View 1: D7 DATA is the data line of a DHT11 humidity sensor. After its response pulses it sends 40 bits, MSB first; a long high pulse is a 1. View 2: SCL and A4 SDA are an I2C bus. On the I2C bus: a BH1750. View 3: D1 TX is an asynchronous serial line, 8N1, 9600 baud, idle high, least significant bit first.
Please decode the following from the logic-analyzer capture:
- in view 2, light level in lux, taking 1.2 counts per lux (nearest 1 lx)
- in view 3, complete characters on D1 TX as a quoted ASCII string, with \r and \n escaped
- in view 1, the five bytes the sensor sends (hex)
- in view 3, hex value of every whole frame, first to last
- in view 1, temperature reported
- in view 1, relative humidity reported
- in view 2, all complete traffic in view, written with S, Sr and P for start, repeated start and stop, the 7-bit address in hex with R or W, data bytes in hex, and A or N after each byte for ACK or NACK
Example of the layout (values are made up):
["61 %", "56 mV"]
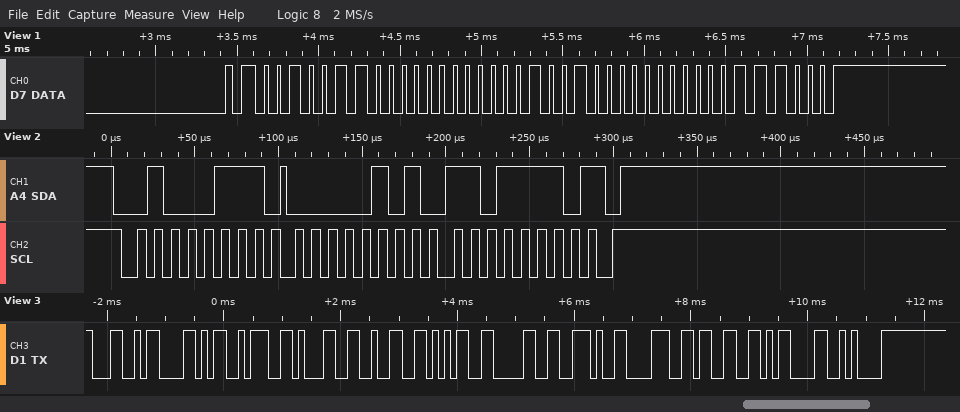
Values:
["1252 lx", "\"LX:1250.83\\r\\n\"", "26 00 12 00 38", "4C 58 3A 31 32 35 30 2E 38 33 0D 0A", "18.0 °C", "38 %", "S 23R A 05 A DE N P"]
